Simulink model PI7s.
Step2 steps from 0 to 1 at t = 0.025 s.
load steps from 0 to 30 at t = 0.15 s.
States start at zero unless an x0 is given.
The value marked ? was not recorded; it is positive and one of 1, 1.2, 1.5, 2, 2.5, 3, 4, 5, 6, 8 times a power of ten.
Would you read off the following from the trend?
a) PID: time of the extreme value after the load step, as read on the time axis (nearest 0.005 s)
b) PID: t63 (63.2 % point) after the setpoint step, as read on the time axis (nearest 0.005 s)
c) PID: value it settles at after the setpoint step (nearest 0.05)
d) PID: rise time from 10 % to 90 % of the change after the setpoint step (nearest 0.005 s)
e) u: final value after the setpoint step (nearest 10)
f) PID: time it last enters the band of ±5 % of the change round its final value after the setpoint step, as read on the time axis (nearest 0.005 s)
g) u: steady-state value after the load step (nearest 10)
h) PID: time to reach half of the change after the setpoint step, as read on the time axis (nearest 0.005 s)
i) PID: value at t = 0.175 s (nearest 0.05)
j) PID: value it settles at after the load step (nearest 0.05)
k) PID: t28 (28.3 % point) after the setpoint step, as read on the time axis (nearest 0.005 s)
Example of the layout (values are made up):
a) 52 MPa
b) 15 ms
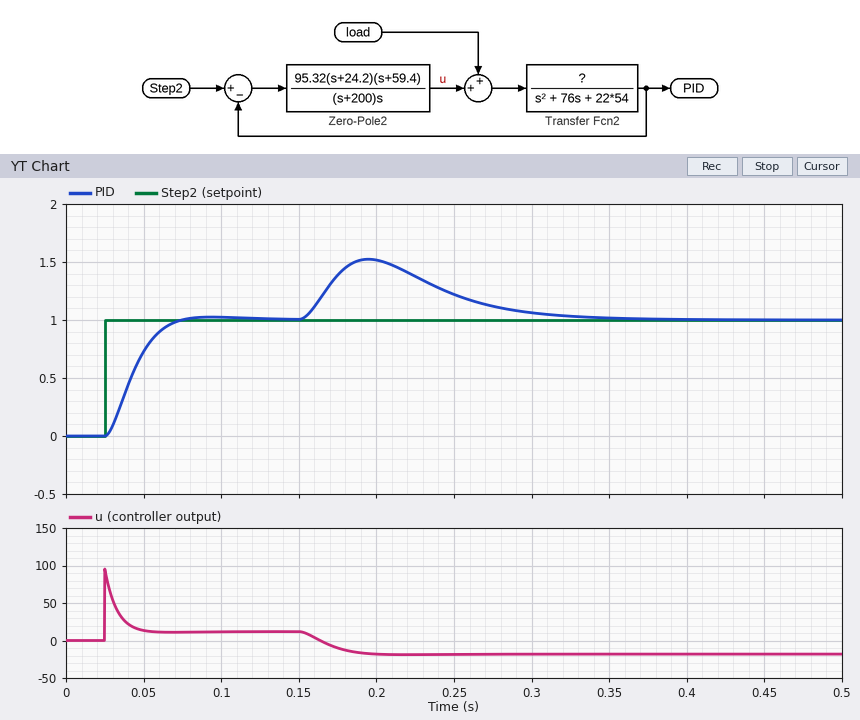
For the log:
a) 0.195 s
b) 0.045 s
c) 1.00
d) 0.030 s
e) 10
f) 0.065 s
g) -20
h) 0.040 s
i) 1.40
j) 1.00
k) 0.035 s
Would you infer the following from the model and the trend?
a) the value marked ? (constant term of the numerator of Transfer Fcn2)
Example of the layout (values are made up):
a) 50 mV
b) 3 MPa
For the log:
a) 100
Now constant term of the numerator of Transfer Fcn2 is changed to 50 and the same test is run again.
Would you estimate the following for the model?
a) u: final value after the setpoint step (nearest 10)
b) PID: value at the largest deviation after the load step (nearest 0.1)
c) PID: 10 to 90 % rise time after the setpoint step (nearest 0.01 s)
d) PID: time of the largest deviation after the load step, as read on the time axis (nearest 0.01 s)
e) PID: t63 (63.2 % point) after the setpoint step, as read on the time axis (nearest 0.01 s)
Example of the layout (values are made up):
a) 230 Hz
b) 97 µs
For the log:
a) 20
b) 1.4
c) 0.06 s
d) 0.21 s
e) 0.06 s
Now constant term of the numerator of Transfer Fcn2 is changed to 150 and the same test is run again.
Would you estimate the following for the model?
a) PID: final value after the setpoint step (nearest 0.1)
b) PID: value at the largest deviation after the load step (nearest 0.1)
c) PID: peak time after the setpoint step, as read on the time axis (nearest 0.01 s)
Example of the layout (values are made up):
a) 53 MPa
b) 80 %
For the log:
a) 1.0
b) 1.6
c) 0.07 s
